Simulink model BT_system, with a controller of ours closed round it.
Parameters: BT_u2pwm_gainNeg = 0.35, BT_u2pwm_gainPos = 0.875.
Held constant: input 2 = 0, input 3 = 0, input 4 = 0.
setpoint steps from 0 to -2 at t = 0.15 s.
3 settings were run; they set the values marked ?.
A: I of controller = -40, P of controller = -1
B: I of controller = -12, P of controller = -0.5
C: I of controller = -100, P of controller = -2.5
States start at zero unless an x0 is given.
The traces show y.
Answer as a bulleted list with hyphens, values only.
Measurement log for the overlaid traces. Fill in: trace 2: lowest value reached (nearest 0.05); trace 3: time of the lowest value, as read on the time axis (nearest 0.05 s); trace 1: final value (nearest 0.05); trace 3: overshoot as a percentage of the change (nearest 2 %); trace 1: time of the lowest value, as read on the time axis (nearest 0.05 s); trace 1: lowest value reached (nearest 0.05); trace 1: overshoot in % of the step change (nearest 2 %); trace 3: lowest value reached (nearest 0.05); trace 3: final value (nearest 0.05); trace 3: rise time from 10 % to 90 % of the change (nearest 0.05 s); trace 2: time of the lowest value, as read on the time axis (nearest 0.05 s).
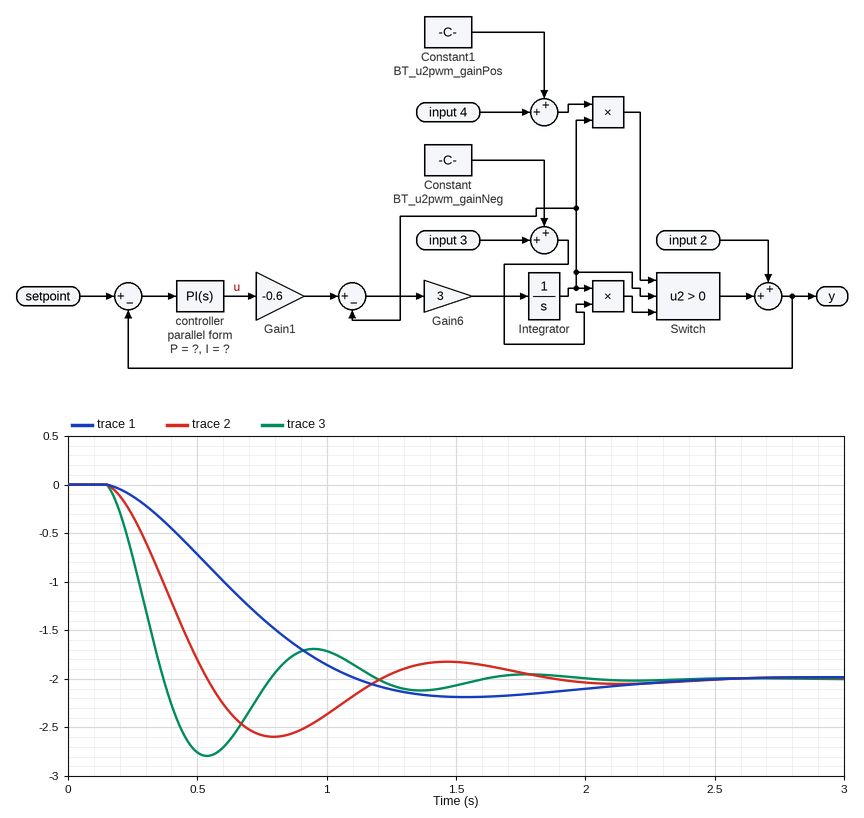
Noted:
- -2.60
- 0.55 s
- -2.00
- 40 %
- 1.55 s
- -2.20
- 10 %
- -2.80
- -2.00
- 0.15 s
- 0.80 s
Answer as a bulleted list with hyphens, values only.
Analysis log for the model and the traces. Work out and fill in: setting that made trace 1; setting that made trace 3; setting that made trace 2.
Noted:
- B
- C
- A
